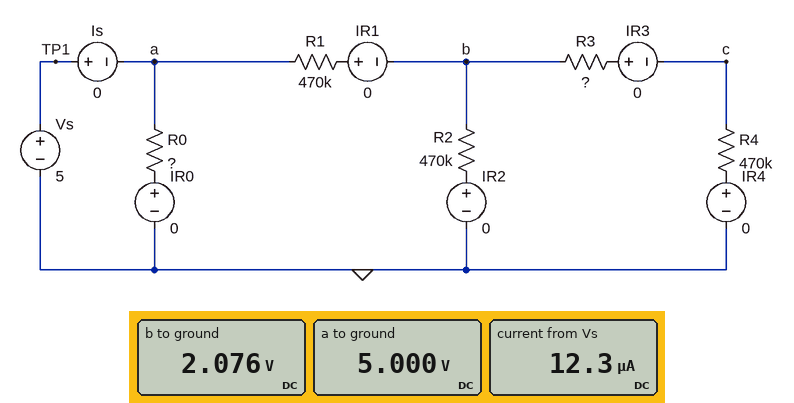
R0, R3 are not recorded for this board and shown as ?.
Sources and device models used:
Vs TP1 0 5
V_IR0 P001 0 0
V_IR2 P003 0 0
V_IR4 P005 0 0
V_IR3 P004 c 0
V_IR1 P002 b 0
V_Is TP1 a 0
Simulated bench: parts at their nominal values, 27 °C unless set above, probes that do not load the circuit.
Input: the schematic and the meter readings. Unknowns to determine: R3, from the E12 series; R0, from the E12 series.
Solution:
680 kΩ
820 kΩ
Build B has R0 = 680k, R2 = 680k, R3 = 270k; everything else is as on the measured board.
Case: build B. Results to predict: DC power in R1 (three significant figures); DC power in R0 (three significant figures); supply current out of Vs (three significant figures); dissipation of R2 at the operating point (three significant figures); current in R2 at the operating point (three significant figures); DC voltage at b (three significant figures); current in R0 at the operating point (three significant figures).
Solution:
17.3 µW
36.8 µW
13.4 µA
6.79 µW
3.16 µA
2.15 V
7.35 µA
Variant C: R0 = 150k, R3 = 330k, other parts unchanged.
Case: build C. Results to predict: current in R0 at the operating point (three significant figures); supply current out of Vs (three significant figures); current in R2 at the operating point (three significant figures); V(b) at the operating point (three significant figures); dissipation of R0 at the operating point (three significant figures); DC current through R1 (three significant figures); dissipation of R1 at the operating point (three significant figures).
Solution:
33.3 µA
39.9 µA
4.11 µA
1.93 V
167 µW
6.53 µA
20.0 µW
